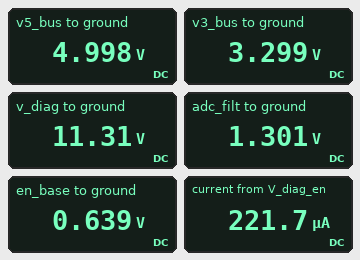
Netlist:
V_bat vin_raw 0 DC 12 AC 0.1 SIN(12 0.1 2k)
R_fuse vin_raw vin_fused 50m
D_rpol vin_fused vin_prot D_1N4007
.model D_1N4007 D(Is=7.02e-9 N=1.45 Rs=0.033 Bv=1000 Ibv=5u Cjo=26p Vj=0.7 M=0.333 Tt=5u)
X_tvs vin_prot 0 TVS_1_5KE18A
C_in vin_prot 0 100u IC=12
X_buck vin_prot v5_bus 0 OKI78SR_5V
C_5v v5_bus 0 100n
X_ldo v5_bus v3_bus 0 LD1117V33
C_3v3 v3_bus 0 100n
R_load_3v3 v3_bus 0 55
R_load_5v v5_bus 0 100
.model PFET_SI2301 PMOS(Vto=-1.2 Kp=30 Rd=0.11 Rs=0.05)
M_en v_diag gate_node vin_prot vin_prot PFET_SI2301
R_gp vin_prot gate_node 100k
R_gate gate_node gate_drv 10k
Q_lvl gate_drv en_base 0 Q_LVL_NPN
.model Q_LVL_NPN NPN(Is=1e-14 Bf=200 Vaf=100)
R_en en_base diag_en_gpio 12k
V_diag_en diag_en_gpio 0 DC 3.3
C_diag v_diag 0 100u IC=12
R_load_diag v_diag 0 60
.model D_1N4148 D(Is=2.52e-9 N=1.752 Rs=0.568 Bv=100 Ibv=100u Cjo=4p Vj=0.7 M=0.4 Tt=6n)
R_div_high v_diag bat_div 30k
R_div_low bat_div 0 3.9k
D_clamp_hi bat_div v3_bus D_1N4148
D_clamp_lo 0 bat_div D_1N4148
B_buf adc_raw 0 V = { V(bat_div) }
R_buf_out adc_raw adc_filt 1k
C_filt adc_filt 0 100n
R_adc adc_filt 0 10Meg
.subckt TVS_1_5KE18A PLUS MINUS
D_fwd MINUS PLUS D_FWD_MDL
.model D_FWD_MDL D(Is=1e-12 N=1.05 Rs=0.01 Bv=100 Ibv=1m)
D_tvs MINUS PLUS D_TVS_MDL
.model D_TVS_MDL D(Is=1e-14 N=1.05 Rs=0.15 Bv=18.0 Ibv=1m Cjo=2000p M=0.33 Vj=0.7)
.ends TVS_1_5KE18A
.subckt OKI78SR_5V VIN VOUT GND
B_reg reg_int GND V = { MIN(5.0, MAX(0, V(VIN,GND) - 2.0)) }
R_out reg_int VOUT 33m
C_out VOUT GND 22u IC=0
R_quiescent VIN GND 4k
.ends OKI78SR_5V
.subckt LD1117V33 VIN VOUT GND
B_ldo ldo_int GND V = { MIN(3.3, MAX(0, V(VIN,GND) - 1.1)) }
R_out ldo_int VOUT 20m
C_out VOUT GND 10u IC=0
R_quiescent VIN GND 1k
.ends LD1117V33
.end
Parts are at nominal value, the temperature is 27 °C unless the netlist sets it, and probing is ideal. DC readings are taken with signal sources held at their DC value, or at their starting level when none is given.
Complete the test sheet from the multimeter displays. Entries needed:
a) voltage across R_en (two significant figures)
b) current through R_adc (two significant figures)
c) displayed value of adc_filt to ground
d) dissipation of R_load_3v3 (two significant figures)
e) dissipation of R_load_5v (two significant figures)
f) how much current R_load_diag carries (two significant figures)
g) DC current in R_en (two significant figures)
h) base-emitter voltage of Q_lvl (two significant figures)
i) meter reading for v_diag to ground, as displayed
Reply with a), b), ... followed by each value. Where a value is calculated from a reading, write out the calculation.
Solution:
a) 3.3 V - 639 mV = 2.7 V
b) (1.301 V) / 10 MΩ = 130 nA
c) 1.301 V
d) (3.299 V)^2 / 55 Ω = 200 mW
e) (4.998 V)^2 / 100 Ω = 250 mW
f) (11.31 V) / 60 Ω = 190 mA
g) (3.3 V - 639 mV) / 12 kΩ = 220 µA
h) 639 mV = 640 mV
i) 11.31 V
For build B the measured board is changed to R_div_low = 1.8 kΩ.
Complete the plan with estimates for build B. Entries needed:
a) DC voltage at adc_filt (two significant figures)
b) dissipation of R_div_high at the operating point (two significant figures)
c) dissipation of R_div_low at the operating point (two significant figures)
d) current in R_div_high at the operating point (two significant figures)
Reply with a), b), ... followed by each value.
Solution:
a) 640 mV
b) 3.8 mW
c) 230 µW
d) 360 µA
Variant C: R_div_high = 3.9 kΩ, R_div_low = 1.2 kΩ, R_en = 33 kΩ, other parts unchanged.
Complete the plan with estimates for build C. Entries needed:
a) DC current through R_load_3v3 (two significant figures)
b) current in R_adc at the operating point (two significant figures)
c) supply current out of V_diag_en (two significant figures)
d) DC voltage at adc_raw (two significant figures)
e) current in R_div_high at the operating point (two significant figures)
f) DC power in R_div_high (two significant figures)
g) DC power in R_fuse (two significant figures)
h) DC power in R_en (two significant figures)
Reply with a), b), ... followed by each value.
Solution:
a) 60 mA
b) 270 nA
c) 81 µA
d) 2.7 V
e) 2.2 mA
f) 19 mW
g) 1.9 mW
h) 220 µW
